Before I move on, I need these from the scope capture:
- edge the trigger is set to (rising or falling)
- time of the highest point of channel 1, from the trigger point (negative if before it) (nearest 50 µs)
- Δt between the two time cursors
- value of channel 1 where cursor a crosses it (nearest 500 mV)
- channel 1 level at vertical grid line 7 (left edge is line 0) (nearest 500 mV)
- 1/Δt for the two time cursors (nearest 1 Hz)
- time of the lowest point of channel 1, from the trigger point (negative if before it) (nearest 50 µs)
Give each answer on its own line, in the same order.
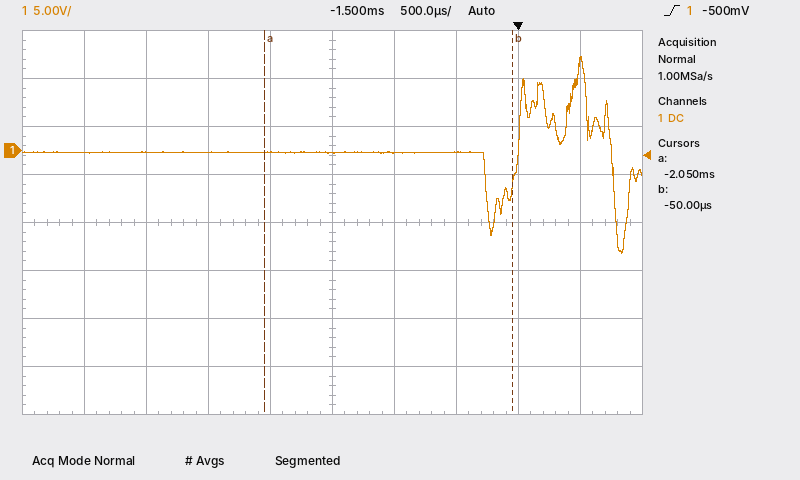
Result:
rising
+500 µs
2.00 ms
0.0 V
0.0 V
500 Hz
+850 µs
